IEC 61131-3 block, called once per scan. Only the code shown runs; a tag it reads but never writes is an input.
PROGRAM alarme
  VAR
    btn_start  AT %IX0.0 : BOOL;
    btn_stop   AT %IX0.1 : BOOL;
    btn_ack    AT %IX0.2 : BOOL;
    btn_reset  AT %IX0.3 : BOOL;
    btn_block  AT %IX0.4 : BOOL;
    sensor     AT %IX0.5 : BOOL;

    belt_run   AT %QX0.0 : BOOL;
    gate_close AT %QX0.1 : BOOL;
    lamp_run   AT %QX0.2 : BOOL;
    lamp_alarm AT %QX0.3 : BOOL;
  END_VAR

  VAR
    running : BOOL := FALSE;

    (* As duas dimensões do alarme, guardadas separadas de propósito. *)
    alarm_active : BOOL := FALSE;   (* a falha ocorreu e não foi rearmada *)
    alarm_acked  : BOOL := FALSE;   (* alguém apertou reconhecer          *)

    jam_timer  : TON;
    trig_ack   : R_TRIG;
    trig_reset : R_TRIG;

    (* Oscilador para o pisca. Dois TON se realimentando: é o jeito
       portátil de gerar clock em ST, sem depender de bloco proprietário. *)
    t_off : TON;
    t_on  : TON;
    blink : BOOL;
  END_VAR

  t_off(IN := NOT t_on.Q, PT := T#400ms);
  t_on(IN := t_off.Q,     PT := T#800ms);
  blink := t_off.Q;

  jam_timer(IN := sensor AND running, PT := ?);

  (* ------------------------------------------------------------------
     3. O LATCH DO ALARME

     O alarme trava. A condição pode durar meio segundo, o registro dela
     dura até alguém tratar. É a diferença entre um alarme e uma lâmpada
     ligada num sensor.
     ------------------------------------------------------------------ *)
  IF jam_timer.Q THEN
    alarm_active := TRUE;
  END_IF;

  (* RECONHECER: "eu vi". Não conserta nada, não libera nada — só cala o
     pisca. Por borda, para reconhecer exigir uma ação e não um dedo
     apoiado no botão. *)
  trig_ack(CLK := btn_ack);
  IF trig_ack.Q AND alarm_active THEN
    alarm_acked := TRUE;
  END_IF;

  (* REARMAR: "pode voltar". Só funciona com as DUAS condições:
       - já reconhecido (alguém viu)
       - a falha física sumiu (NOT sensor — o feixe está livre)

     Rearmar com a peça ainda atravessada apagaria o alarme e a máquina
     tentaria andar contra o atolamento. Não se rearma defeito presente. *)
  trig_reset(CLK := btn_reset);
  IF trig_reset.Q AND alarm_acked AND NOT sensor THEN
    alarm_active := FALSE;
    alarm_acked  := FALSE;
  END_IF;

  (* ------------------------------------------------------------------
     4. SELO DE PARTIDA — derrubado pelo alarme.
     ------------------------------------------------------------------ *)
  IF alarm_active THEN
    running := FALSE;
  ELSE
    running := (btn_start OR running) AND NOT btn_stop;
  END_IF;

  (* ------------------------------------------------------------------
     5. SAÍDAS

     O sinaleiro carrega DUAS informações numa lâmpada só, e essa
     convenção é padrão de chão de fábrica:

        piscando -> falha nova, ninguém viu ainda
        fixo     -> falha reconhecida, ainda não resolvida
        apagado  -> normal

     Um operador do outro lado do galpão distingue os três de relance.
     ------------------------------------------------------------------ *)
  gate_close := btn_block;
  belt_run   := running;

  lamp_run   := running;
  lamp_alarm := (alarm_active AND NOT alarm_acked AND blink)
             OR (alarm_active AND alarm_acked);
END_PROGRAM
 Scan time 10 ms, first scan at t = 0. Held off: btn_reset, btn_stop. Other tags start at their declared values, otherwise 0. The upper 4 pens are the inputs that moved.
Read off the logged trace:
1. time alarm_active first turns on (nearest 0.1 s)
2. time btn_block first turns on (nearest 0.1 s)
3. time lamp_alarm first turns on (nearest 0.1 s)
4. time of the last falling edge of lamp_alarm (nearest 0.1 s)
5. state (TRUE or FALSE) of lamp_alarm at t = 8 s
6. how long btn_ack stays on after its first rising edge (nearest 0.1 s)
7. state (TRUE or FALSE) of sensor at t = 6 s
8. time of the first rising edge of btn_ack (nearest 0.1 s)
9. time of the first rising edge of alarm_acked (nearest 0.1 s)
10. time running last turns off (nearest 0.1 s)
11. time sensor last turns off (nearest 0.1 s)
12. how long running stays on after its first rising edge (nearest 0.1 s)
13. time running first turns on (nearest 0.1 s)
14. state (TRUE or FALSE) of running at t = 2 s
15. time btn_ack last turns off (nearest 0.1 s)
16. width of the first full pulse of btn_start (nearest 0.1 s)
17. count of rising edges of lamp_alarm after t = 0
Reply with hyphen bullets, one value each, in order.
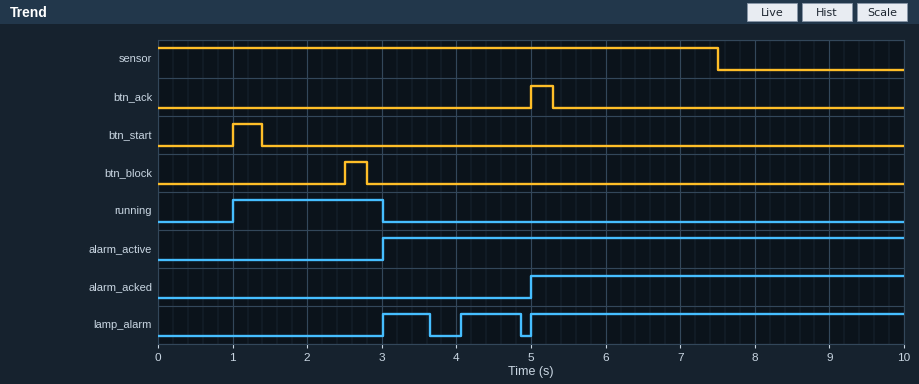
- 3.0 s
- 2.5 s
- 3.0 s
- 4.9 s
- TRUE
- 0.3 s
- TRUE
- 5.0 s
- 5.0 s
- 3.0 s
- 7.5 s
- 2.0 s
- 1.0 s
- TRUE
- 5.3 s
- 0.4 s
- 3
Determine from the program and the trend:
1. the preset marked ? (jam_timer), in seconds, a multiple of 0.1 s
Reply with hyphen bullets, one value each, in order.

- 2.0 s
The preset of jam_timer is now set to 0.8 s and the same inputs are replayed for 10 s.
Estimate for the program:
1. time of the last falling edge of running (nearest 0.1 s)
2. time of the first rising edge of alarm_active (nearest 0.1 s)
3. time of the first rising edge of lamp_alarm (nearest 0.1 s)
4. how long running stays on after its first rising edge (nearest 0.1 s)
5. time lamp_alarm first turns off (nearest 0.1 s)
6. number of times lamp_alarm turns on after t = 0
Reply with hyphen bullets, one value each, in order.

- 1.8 s
- 1.8 s
- 1.8 s
- 0.8 s
- 2.4 s
- 4
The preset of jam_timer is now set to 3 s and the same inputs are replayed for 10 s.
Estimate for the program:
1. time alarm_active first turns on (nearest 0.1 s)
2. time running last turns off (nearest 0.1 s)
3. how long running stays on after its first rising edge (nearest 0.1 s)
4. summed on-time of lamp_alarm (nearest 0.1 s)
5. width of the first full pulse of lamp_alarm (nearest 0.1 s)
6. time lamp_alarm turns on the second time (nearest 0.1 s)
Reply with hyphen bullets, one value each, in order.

- 4.0 s
- 4.0 s
- 3.0 s
- 5.8 s
- 0.8 s
- 5.0 s
